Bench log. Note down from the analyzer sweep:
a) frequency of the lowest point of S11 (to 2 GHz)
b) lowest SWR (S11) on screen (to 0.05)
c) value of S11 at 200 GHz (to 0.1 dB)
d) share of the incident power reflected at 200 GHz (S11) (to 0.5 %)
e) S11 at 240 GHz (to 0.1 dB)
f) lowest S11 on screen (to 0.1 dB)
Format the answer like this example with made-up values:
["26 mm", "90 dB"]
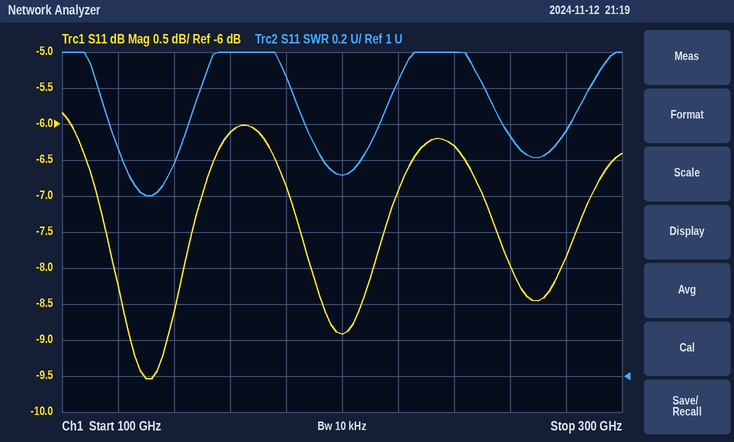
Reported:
["130 GHz", "2.00", "-8.9 dB", "13.0 %", "-6.3 dB", "-9.5 dB"]
